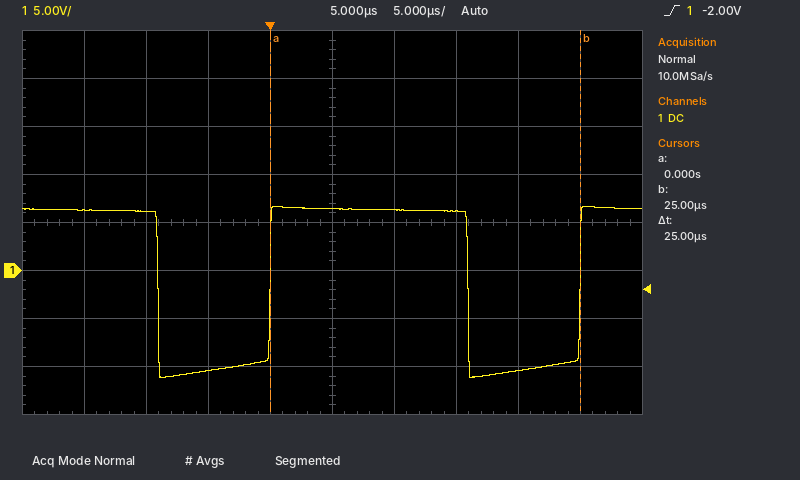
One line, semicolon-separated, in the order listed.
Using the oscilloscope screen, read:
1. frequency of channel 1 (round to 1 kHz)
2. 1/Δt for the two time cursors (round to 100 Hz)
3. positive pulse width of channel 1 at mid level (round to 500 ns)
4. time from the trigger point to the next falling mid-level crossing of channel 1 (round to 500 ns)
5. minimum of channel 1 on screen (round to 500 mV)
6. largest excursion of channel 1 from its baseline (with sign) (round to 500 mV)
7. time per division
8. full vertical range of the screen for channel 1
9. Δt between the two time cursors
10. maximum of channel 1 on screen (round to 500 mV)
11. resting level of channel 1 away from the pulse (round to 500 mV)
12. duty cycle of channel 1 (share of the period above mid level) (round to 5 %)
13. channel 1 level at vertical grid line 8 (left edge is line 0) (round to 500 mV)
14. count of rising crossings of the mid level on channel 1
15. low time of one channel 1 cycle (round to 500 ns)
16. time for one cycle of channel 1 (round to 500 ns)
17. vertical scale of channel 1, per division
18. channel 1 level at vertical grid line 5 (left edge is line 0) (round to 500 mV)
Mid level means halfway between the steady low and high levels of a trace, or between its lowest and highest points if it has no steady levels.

40 kHz; 40.0 kHz; 16.0 µs; 16.0 µs; -11.0 V; -17.5 V; 5 µs; 40 V; 25 µs; 6.5 V; 6.5 V; 65 %; -10.5 V; 2; 9.0 µs; 25.0 µs; 5 V; 6.5 V
